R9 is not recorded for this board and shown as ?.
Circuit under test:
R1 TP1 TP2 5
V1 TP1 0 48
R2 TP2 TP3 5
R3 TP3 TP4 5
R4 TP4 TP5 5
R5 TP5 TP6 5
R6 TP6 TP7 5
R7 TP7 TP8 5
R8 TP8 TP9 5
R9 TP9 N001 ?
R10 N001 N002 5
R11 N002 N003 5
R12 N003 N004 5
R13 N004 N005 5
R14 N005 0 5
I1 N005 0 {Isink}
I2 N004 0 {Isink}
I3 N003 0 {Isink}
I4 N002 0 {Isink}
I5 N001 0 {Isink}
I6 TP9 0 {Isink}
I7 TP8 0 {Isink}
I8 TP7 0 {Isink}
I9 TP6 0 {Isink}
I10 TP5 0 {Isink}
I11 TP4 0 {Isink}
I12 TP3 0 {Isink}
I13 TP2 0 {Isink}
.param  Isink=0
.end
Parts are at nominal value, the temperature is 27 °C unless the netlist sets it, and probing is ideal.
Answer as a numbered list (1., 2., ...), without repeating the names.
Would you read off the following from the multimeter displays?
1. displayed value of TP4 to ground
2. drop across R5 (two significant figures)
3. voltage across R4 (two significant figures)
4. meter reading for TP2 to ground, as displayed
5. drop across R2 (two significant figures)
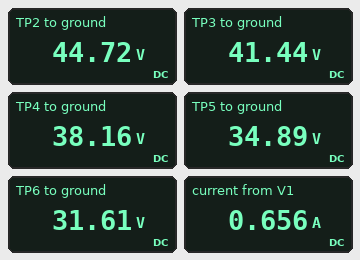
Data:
1. 38.16 V
2. 3.3 V
3. 3.3 V
4. 44.72 V
5. 3.3 V
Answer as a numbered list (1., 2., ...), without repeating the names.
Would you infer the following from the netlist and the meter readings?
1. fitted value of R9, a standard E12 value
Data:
1. 8.2 Ω
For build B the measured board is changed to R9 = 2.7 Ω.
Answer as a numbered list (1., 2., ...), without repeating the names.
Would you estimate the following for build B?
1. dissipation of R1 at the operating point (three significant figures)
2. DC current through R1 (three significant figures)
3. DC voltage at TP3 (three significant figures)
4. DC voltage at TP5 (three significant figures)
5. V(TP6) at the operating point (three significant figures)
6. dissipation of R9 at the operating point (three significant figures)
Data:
1. 2.51 W
2. 709 mA
3. 40.9 V
4. 33.8 V
5. 30.3 V
6. 1.36 W
